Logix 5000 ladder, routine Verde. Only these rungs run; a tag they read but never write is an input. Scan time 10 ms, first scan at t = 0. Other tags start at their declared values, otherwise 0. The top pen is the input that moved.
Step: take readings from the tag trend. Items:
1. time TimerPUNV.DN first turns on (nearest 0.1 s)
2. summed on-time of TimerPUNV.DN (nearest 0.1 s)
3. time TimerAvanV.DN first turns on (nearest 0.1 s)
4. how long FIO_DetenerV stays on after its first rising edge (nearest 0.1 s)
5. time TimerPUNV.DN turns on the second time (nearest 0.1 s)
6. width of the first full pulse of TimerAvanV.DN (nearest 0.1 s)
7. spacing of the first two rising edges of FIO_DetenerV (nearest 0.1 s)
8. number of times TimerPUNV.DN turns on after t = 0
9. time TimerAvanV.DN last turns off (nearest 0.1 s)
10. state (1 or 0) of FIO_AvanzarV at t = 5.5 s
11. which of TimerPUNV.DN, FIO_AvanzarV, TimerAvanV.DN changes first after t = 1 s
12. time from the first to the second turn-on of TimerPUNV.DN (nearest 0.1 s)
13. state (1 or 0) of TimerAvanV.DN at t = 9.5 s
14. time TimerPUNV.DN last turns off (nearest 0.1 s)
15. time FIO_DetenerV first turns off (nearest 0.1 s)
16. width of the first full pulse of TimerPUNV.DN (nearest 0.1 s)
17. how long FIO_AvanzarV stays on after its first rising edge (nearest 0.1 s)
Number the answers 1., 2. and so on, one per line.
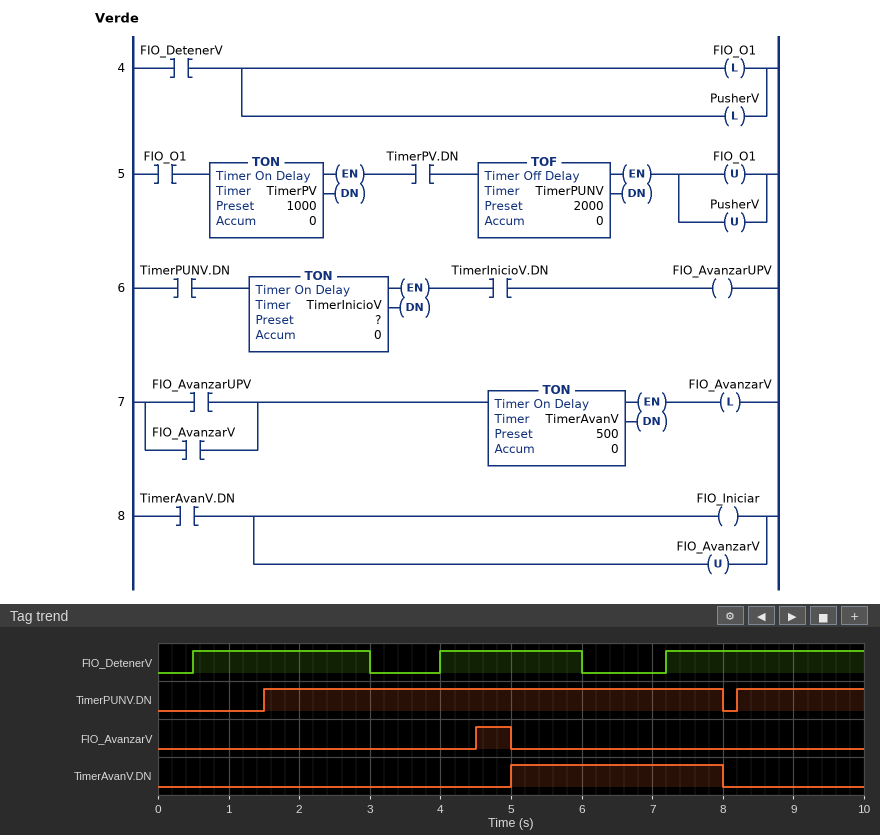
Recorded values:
1. 1.5 s
2. 8.3 s
3. 5.0 s
4. 2.5 s
5. 8.2 s
6. 3.0 s
7. 3.5 s
8. 2
9. 8.0 s
10. 0
11. TimerPUNV.DN
12. 6.7 s
13. 0
14. 8.0 s
15. 3.0 s
16. 6.5 s
17. 0.5 s
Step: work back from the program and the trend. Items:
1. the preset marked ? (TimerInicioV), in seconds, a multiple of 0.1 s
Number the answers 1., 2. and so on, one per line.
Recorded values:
1. 3.0 s
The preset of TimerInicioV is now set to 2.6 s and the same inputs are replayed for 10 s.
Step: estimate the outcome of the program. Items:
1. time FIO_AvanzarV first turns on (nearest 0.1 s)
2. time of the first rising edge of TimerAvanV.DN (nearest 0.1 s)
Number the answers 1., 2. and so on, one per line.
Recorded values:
1. 4.1 s
2. 4.6 s
